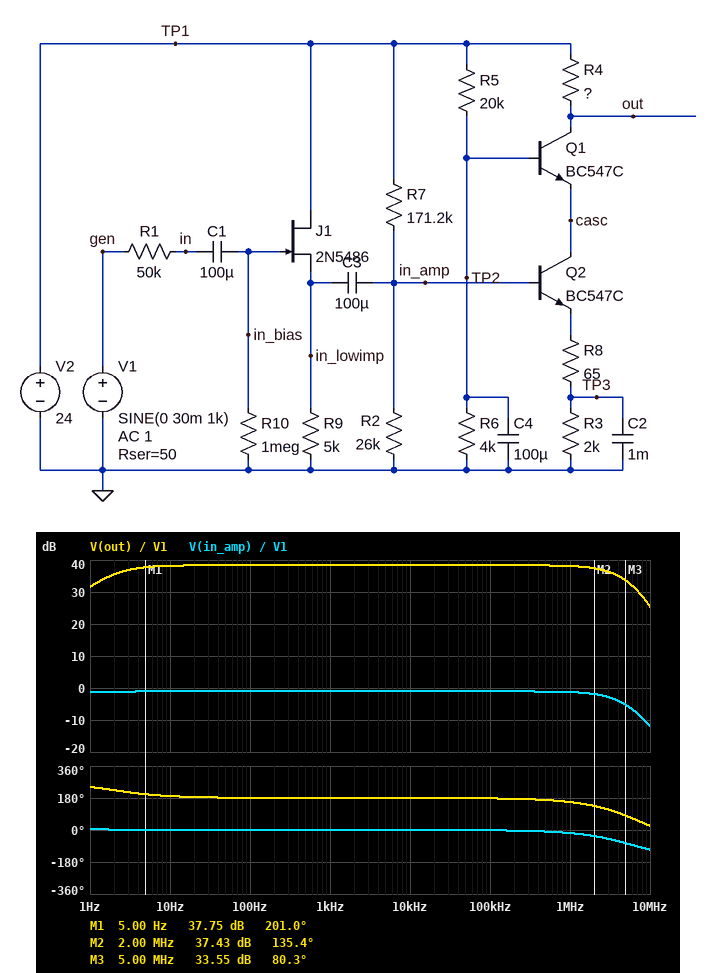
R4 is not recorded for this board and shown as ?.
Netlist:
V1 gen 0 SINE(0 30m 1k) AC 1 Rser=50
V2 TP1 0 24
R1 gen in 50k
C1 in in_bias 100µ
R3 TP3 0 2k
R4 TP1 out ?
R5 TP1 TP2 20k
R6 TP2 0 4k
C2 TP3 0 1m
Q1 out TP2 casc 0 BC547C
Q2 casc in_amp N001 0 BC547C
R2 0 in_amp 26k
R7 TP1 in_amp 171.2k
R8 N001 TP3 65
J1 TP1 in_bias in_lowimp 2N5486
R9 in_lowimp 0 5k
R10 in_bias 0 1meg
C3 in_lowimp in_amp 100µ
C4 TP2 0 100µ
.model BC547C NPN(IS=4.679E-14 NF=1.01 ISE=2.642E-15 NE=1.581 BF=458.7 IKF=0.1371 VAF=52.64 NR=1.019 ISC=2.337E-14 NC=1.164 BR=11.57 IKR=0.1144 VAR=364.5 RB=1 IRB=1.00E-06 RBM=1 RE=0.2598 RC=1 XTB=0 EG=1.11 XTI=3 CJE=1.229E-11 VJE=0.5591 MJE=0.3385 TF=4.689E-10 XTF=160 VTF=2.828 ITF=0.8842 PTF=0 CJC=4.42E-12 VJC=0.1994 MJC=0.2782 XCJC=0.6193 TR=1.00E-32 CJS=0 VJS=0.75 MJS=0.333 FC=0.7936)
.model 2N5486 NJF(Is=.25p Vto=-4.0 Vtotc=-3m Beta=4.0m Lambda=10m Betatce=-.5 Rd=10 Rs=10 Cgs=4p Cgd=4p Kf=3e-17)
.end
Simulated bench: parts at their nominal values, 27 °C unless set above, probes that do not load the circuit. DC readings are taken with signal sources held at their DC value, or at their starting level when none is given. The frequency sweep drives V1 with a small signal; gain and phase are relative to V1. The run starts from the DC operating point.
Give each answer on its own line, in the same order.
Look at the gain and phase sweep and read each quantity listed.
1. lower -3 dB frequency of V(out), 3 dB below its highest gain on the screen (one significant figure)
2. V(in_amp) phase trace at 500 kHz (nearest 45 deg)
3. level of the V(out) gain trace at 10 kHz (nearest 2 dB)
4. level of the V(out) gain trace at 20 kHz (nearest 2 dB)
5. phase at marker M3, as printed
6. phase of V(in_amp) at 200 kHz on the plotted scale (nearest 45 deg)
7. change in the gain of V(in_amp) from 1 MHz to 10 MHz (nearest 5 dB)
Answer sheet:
2 Hz
0 deg
38 dB
38 dB
80.3 deg
0 deg
-10 dB
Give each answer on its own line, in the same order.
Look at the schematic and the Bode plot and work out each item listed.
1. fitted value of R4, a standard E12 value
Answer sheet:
8.2 kΩ
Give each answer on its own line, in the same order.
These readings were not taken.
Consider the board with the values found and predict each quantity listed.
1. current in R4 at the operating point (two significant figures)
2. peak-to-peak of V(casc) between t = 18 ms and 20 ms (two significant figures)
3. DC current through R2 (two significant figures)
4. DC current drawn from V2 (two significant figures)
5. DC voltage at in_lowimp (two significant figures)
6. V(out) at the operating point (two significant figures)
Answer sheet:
1.2 mA
16 mV
120 µA
3.0 mA
3.6 V
14 V
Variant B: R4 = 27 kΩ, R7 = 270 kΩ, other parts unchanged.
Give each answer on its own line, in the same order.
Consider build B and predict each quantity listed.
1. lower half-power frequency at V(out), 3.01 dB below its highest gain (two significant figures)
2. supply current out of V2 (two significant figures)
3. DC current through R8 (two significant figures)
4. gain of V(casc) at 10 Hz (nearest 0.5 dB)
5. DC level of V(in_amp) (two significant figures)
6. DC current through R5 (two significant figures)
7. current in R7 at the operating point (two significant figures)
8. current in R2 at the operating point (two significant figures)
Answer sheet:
1.7 Hz
2.5 mA
710 µA
-7.5 dB
2.1 V
1.0 mA
81 µA
80 µA
